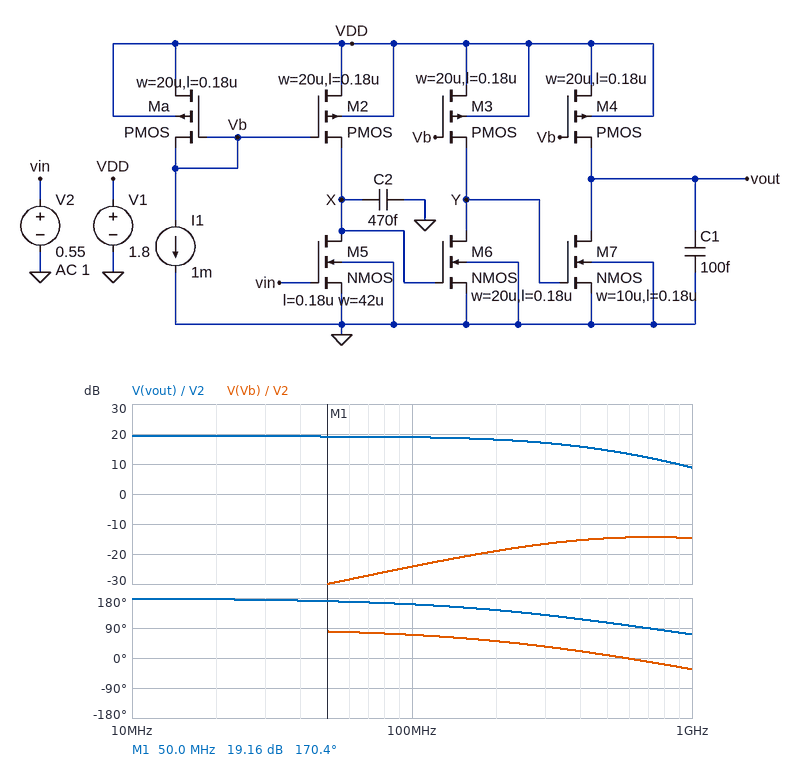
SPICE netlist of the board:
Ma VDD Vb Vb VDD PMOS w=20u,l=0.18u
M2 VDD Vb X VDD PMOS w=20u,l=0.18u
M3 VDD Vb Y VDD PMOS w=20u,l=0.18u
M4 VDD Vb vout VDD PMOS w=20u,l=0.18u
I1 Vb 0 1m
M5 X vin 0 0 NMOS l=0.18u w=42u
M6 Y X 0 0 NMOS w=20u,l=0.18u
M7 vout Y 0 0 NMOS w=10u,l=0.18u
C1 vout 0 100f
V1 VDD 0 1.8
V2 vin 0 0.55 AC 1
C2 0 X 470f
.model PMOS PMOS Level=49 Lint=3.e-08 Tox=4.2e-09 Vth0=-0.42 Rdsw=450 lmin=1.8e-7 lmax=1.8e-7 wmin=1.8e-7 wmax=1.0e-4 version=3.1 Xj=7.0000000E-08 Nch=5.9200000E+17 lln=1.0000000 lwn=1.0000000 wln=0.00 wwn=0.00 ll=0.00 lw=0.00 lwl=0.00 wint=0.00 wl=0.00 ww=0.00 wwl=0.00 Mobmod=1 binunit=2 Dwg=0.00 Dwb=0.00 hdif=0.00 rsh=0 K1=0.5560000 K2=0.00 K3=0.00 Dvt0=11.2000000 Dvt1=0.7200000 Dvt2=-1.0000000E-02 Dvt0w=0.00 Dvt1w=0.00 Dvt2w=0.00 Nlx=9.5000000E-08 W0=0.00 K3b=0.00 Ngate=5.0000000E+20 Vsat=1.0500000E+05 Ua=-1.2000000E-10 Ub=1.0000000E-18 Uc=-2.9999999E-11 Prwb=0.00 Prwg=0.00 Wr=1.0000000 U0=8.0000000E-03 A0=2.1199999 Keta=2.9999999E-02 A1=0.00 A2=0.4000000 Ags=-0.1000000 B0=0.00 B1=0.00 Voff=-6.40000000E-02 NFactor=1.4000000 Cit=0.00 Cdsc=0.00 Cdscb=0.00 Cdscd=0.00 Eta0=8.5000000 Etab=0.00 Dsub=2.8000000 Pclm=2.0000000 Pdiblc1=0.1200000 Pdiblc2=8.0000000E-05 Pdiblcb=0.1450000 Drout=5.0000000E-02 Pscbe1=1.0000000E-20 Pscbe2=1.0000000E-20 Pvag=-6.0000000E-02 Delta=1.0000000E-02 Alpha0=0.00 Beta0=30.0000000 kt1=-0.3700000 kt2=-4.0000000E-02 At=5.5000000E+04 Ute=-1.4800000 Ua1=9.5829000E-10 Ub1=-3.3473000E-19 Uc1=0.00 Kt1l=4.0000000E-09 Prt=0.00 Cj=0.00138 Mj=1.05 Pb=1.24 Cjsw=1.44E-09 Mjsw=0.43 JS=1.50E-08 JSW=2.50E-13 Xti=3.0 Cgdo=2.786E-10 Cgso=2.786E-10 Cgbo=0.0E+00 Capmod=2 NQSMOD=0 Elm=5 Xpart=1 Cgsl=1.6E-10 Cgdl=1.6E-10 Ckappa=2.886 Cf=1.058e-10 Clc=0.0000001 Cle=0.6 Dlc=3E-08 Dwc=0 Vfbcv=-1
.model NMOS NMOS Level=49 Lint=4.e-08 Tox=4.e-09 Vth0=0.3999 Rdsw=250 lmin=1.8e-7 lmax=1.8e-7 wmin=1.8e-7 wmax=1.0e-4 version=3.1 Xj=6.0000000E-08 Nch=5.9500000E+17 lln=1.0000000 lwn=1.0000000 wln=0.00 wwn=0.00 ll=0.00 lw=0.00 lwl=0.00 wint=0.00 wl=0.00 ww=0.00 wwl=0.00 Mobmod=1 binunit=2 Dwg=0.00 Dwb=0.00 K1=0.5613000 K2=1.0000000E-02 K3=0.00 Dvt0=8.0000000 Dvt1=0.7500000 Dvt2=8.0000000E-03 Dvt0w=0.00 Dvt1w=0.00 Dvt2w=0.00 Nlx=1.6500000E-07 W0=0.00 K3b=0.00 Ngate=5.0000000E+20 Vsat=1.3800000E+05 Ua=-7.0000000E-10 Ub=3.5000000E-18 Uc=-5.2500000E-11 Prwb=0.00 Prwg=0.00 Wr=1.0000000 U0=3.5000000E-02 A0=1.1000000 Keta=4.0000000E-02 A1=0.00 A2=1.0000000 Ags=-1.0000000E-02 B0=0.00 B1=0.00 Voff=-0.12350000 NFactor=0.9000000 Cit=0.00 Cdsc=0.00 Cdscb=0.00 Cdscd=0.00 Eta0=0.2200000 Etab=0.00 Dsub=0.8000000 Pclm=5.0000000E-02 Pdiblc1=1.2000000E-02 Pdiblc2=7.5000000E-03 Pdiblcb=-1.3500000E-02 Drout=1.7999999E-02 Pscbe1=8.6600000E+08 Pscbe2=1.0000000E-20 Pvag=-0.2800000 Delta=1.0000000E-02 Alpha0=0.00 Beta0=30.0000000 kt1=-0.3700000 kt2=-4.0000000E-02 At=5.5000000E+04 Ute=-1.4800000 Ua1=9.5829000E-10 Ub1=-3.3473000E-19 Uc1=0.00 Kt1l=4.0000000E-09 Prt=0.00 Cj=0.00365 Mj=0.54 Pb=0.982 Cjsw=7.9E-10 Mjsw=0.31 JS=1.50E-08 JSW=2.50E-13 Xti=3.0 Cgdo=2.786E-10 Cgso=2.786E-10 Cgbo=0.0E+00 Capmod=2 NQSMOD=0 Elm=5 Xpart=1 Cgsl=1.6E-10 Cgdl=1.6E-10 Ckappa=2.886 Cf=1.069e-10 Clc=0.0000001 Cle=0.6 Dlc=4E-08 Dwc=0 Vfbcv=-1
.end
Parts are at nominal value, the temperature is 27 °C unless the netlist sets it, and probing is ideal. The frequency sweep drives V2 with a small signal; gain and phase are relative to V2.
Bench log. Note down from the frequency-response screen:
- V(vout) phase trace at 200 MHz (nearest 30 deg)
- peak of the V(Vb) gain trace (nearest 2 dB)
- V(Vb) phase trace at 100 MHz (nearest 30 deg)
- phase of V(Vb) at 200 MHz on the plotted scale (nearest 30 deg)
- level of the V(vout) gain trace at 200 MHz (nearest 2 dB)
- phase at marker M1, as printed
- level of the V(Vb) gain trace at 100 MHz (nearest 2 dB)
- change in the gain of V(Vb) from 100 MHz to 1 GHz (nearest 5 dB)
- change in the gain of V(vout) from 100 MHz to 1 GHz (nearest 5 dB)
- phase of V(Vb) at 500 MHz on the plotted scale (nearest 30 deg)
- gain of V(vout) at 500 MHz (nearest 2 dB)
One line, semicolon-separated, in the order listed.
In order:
150 deg; -14 dB; 60 deg; 60 deg; 18 dB; 170.4 deg; -24 dB; 10 dB; -10 dB; 0 deg; 14 dB
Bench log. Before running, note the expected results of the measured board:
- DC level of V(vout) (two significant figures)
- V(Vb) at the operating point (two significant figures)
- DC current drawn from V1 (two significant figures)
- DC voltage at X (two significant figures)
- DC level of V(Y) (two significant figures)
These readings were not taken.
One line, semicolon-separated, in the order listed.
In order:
150 mV; 1.1 V; 4.6 mA; 560 mV; 1.1 V
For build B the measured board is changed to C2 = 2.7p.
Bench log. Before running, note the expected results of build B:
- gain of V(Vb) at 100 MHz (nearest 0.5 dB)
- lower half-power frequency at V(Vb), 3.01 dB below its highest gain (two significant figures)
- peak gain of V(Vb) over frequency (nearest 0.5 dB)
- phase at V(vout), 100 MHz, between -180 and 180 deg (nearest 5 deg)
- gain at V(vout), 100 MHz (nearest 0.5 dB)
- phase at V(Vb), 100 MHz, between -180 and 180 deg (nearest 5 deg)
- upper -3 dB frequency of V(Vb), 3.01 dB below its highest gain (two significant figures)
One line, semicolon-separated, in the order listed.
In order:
-28.0 dB; 75 MHz; -26.0 dB; 125 deg; 15.5 dB; 35 deg; 1.5 GHz
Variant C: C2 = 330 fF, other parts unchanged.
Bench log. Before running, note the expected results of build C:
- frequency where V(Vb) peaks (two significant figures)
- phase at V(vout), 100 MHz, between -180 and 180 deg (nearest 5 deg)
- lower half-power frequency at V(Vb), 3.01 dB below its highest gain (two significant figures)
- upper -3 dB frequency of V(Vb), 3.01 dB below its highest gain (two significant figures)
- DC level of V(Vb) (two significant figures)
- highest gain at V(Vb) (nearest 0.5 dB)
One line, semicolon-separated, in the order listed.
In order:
800 MHz; 165 deg; 310 MHz; 2.0 GHz; 1.1 V; -12.5 dB
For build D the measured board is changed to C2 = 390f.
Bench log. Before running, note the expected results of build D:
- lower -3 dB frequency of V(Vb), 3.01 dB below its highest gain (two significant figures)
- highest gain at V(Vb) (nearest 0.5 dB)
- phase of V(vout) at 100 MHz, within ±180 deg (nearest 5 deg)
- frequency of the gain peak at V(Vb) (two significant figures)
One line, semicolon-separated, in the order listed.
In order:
290 MHz; -13.5 dB; 165 deg; 760 MHz
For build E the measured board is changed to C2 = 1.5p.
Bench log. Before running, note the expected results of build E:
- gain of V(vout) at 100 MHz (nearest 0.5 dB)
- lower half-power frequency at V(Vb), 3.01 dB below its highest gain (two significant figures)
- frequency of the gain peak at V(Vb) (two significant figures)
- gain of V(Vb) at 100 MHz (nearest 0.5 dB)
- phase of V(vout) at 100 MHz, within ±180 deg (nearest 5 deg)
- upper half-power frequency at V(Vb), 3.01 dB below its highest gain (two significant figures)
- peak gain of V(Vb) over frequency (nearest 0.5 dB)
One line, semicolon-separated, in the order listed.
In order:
17.5 dB; 120 MHz; 450 MHz; -25.5 dB; 140 deg; 1.6 GHz; -21.5 dB
